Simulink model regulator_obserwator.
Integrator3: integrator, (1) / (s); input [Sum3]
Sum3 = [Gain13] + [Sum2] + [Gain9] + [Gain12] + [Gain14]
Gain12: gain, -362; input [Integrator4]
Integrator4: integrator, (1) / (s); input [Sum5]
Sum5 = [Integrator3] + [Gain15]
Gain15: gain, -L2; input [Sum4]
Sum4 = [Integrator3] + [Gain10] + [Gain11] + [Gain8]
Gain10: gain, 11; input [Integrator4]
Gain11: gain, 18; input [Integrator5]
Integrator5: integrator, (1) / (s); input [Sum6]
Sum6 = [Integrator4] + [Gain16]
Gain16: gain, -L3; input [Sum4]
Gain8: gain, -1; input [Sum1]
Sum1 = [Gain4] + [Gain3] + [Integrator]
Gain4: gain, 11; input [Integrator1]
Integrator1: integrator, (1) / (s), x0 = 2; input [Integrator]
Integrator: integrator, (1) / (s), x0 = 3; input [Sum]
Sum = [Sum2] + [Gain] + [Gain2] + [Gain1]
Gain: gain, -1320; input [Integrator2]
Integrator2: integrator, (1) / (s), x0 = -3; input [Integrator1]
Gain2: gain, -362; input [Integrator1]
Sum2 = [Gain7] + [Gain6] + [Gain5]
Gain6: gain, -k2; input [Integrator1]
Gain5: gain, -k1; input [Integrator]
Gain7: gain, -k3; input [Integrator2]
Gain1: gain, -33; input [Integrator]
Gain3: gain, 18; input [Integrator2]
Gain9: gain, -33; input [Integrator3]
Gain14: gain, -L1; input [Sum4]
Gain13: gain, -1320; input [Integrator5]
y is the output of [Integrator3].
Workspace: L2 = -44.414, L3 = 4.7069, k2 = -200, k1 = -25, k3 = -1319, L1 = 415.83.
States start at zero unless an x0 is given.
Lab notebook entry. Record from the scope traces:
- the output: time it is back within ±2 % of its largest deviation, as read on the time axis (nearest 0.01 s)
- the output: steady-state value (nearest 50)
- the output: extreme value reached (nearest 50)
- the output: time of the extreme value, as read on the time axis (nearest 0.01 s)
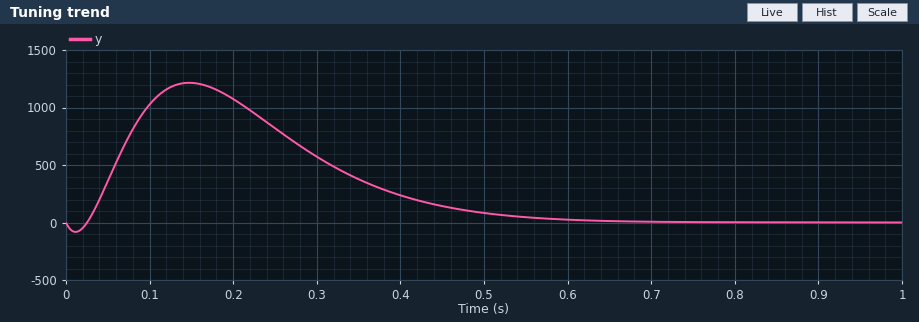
0.60 s
0
1200
0.15 s
